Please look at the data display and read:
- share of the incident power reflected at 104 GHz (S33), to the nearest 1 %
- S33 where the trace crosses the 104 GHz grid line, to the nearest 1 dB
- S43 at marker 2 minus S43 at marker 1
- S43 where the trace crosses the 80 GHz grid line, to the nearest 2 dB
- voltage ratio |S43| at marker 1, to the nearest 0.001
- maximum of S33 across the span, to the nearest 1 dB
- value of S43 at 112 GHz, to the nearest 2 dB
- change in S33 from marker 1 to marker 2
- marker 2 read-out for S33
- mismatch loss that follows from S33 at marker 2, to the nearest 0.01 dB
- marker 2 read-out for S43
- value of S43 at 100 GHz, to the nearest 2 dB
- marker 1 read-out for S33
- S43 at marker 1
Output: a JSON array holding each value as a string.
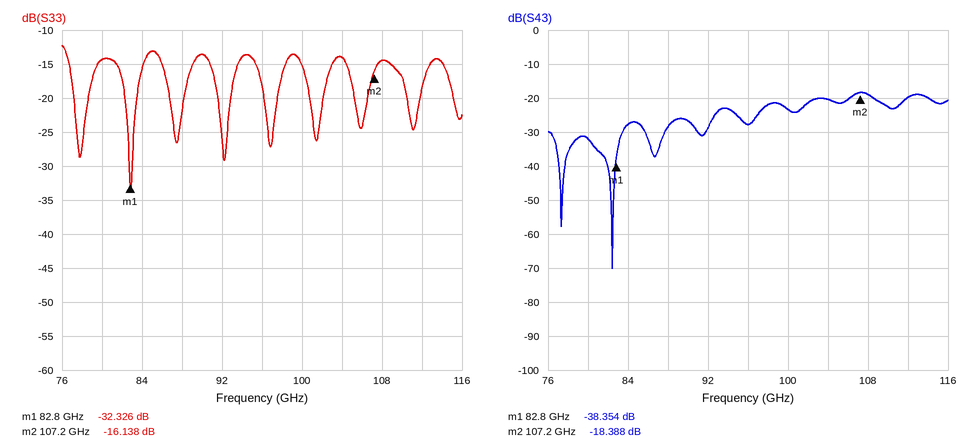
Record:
["4 %", "-14 dB", "19.966 dB", "-32 dB", "0.012", "-12 dB", "-20 dB", "16.188 dB", "-16.138 dB", "0.11 dB", "-18.388 dB", "-24 dB", "-32.326 dB", "-38.354 dB"]
